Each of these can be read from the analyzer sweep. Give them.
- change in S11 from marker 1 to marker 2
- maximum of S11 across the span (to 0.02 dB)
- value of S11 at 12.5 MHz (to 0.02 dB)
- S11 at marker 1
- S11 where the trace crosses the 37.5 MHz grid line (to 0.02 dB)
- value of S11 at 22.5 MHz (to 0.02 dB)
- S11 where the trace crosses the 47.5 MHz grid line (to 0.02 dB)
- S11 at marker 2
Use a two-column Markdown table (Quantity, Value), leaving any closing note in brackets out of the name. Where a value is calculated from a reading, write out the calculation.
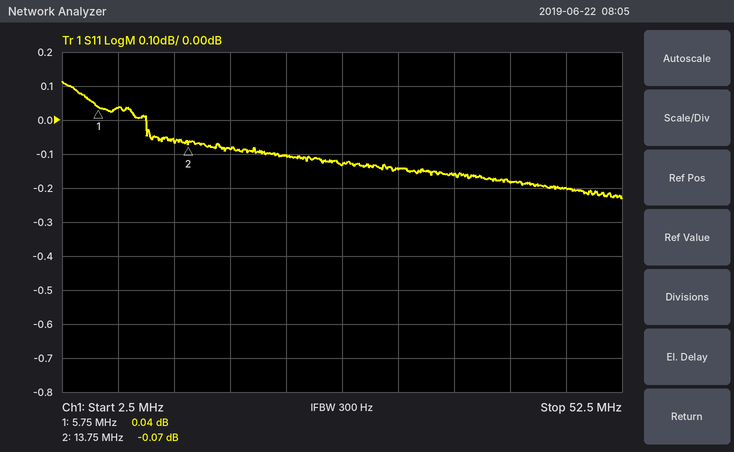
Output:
| Quantity | Value |
|---|---|
| change in S11 from marker 1 to marker 2 | -0.07 − (0.04) = -0.11 dB |
| maximum of S11 across the span | 0.12 dB |
| value of S11 at 12.5 MHz | -0.06 dB |
| S11 at marker 1 | 0.04 dB |
| S11 where the trace crosses the 37.5 MHz grid line | -0.16 dB |
| value of S11 at 22.5 MHz | -0.10 dB |
| S11 where the trace crosses the 47.5 MHz grid line | -0.20 dB |
| S11 at marker 2 | -0.07 dB |
